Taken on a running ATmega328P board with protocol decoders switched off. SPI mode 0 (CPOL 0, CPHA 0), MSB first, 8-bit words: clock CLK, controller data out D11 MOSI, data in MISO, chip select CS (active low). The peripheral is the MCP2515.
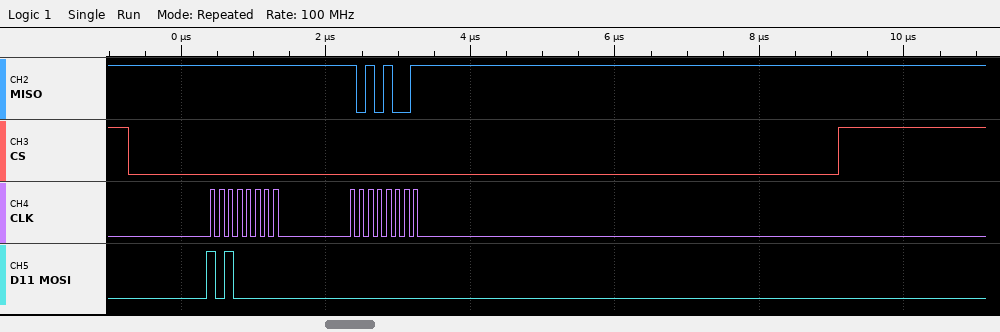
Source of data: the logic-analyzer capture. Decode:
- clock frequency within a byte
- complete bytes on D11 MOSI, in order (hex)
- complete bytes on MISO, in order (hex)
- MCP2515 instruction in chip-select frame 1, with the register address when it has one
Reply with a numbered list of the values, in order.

1. 8 MHz
2. A0 00
3. FF A9
4. READ STATUS
